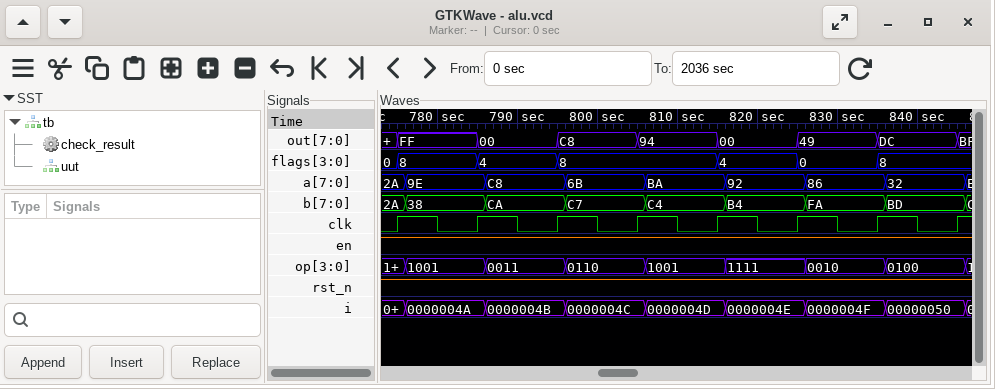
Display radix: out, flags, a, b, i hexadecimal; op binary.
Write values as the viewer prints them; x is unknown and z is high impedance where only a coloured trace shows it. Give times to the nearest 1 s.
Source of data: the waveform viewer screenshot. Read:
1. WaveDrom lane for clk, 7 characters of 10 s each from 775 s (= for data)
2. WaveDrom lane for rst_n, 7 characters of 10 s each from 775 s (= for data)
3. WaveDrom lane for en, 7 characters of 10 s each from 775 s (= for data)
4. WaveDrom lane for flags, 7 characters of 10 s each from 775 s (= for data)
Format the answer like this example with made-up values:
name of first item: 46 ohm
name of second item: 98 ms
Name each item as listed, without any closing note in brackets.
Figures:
WaveDrom lane for clk, 7 characters of 10 s each from 775 s: {name: 'clk', wave: 'p......'}
WaveDrom lane for rst_n, 7 characters of 10 s each from 775 s: {name: 'rst_n', wave: '1......'}
WaveDrom lane for en, 7 characters of 10 s each from 775 s: {name: 'en', wave: '1......'}
WaveDrom lane for flags, 7 characters of 10 s each from 775 s: {name: 'flags', wave: '===.===', data: '8 4 8 4 0 8'}
